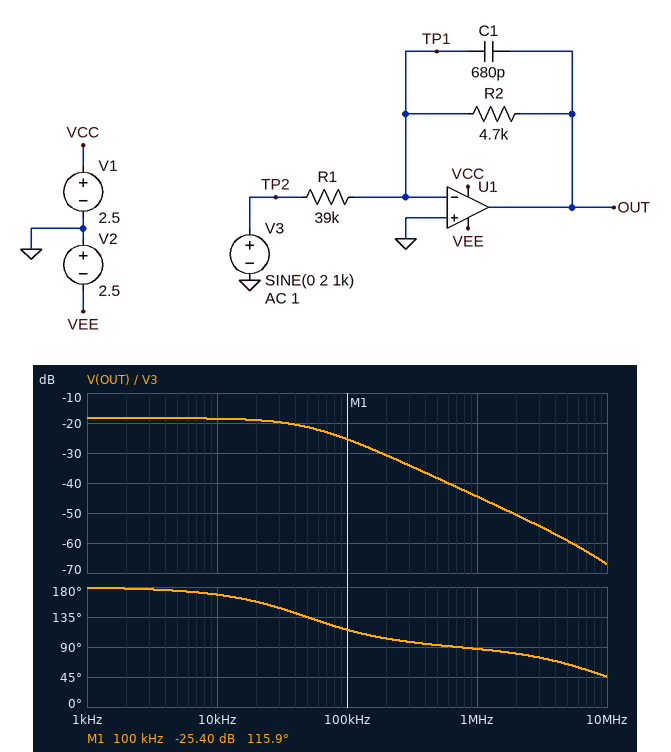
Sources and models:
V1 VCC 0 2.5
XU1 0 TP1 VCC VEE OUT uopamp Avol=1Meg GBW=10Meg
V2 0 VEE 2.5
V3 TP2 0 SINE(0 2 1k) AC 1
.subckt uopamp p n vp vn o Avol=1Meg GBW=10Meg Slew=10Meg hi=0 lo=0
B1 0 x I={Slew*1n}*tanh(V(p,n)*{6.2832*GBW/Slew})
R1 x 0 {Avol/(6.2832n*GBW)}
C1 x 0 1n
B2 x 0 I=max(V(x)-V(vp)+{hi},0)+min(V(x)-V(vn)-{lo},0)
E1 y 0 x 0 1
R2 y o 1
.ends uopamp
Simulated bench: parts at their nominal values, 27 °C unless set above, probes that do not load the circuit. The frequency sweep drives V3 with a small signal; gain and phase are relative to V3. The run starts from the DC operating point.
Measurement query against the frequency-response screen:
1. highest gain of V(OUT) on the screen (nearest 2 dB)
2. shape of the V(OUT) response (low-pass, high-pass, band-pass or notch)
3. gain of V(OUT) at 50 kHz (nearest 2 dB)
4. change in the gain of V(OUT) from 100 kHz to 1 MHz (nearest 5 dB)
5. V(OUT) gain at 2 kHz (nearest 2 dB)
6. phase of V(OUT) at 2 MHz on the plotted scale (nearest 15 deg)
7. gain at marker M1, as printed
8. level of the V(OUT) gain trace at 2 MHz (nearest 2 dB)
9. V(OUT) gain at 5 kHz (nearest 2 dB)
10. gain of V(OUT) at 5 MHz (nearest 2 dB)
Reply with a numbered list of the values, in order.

1. -18 dB
2. low-pass
3. -22 dB
4. -20 dB
5. -18 dB
6. 75 deg
7. -25.40 dB
8. -50 dB
9. -18 dB
10. -60 dB
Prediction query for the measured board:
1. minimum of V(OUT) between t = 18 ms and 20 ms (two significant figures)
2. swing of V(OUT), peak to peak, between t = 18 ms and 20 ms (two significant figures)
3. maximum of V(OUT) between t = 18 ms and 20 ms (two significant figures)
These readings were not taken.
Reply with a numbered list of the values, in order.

1. -240 mV
2. 480 mV
3. 240 mV
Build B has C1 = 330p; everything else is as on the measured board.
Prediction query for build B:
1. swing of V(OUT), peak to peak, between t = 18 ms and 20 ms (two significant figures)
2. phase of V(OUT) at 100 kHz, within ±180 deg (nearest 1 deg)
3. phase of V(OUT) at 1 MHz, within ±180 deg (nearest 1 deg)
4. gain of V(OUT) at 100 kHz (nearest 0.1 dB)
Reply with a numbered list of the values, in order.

1. 480 mV
2. 135 deg
3. 90 deg
4. -21.3 dB
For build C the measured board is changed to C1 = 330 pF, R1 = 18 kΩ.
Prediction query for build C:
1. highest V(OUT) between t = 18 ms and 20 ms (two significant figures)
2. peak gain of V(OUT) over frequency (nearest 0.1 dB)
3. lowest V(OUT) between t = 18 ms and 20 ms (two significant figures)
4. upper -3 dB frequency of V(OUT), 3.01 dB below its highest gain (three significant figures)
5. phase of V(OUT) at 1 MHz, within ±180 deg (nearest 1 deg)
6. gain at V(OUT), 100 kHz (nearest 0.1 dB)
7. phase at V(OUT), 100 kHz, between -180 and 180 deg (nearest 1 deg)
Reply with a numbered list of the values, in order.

1. 520 mV
2. -11.7 dB
3. -520 mV
4. 102 kHz
5. 90 deg
6. -14.6 dB
7. 135 deg
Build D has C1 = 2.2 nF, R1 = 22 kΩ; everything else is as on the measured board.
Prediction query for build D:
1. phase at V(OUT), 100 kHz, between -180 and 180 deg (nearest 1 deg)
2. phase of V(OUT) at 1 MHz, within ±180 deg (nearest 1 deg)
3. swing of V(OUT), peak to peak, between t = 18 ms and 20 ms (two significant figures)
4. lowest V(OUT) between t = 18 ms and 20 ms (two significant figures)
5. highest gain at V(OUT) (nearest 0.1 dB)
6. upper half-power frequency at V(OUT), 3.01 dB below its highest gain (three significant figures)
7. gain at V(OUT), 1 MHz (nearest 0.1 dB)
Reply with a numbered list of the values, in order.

1. 98 deg
2. 85 deg
3. 850 mV
4. -430 mV
5. -13.4 dB
6. 15.4 kHz
7. -49.7 dB
